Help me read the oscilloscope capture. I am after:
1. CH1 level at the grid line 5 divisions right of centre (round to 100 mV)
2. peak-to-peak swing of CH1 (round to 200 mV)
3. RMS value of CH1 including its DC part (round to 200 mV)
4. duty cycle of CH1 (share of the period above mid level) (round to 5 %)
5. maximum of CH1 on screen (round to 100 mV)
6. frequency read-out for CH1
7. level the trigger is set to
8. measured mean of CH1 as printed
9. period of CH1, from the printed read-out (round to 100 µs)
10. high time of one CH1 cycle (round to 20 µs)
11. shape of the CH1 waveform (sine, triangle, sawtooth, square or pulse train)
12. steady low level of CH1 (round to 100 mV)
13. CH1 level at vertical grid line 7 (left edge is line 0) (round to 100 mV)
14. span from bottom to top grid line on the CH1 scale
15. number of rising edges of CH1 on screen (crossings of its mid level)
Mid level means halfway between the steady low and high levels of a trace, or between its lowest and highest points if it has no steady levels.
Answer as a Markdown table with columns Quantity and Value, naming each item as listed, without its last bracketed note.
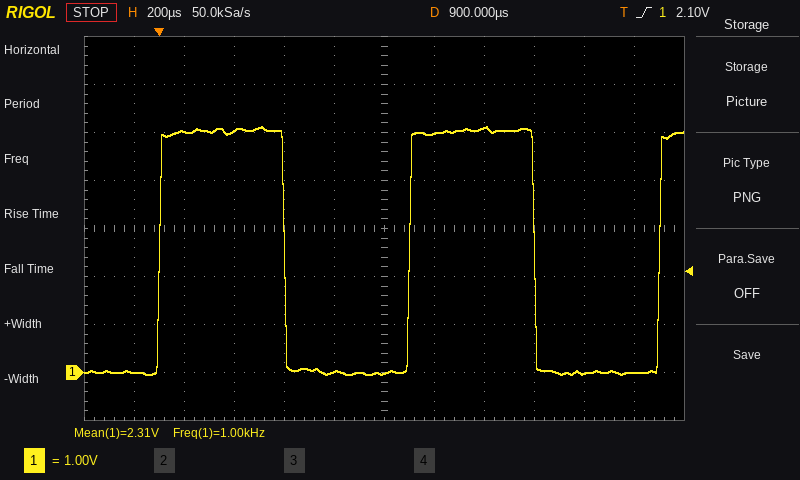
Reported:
| Quantity | Value |
|---|---|
| CH1 level at the grid line 5 divisions right of centre | 0.0 V |
| peak-to-peak swing of CH1 | 5.2 V |
| RMS value of CH1 including its DC part | 3.6 V |
| duty cycle of CH1 (share of the period above mid level) | 50 % |
| maximum of CH1 on screen | 5.1 V |
| frequency read-out for CH1 | 1.00 kHz |
| level the trigger is set to | 2.10 V |
| measured mean of CH1 as printed | 2.31 V |
| period of CH1, from the printed read-out | 1.0 ms |
| high time of one CH1 cycle | 500 µs |
| shape of the CH1 waveform | square |
| steady low level of CH1 | 0.0 V |
| CH1 level at vertical grid line 7 (left edge is line 0) | 5.0 V |
| span from bottom to top grid line on the CH1 scale | 8 V |
| number of rising edges of CH1 on screen | 3 |
